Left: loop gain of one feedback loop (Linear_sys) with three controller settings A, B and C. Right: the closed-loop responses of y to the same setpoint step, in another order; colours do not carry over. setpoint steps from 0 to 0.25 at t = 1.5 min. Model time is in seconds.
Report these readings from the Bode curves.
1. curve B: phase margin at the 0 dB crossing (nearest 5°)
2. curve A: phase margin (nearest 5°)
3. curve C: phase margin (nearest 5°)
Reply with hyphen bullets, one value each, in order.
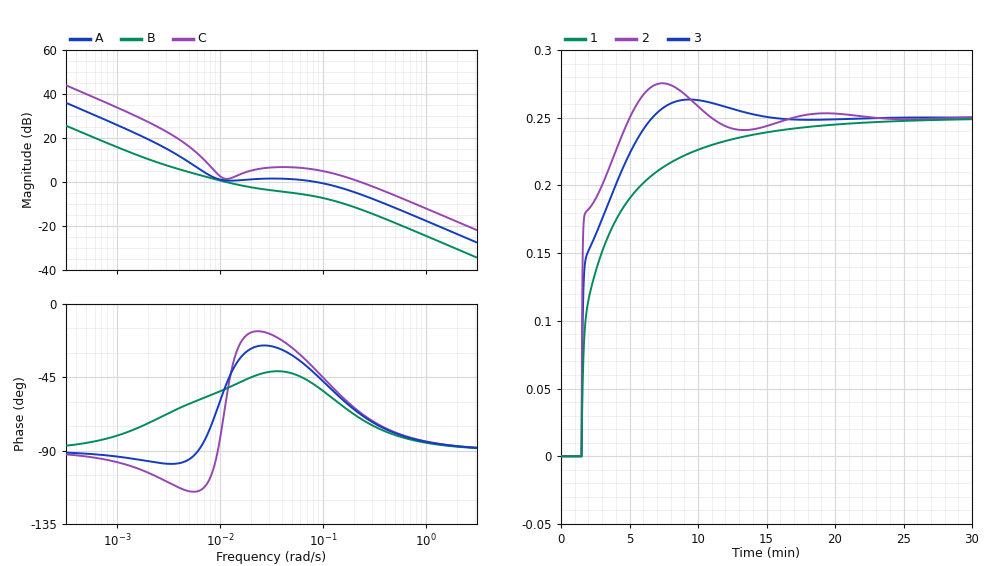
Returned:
- 130°
- 135°
- 115°
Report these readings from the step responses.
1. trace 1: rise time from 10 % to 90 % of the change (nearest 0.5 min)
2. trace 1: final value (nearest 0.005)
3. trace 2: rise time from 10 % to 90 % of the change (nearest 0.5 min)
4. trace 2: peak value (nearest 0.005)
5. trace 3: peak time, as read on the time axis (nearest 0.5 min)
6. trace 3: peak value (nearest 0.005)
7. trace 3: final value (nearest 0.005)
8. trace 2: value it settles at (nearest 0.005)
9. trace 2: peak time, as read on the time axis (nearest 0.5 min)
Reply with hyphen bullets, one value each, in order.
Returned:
- 8.0 min
- 0.250
- 2.5 min
- 0.275
- 9.5 min
- 0.265
- 0.250
- 0.250
- 7.5 min
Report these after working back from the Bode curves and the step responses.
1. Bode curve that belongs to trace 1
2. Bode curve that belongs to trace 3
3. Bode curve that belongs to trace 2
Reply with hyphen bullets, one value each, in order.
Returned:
- B
- A
- C
